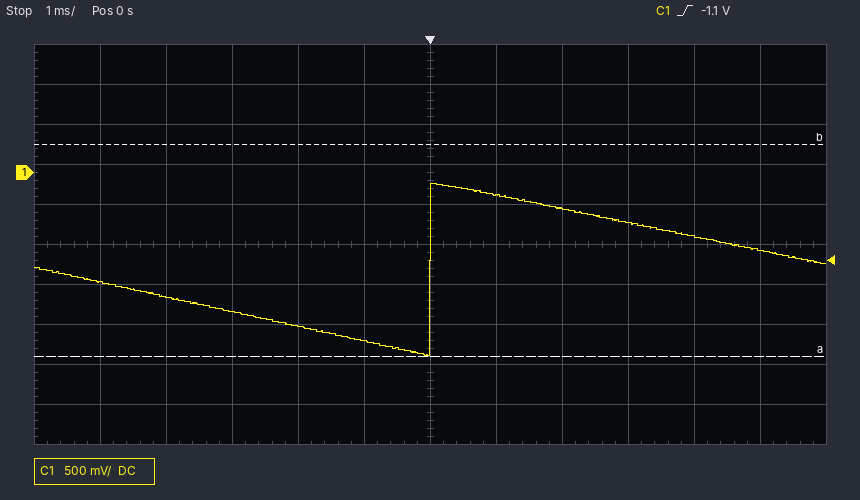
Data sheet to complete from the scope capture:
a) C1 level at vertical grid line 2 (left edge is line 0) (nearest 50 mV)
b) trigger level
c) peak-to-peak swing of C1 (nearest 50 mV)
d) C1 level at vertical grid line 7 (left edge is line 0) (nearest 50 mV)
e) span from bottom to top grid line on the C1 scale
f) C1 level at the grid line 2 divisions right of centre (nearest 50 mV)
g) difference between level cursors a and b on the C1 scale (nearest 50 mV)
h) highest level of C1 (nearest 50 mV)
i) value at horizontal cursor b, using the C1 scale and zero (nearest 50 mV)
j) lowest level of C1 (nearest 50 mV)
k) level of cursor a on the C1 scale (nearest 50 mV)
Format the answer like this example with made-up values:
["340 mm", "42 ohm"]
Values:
["-1.55 V", "-1.1 V", "2.15 V", "-300 mV", "5 V", "-450 mV", "2.65 V", "-150 mV", "350 mV", "-2.30 V", "-2.30 V"]
